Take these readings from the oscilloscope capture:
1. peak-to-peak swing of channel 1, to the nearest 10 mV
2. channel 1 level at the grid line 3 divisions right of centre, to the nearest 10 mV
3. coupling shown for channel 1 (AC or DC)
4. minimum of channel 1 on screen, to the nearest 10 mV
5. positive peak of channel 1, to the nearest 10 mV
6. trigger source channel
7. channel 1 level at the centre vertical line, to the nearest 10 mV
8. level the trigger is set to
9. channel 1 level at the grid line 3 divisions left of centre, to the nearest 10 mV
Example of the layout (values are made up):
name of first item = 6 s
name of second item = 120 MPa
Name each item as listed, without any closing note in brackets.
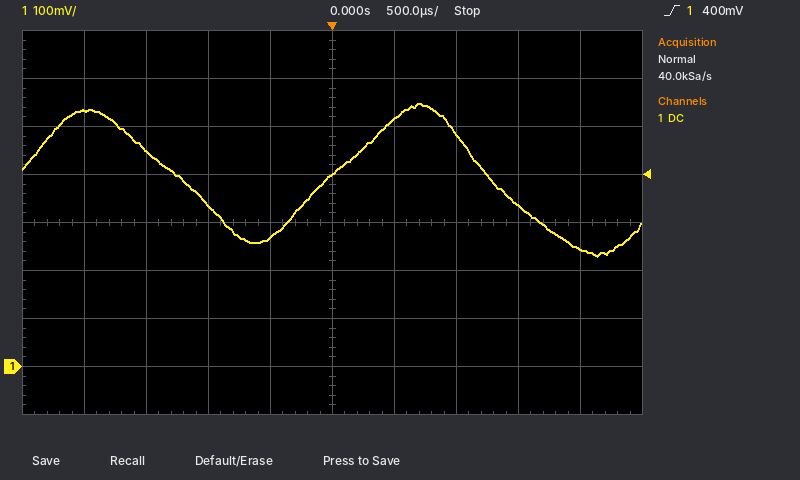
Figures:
peak-to-peak swing of channel 1, to the nearest 10 mV = 320 mV
channel 1 level at the grid line 3 divisions right of centre, to the nearest 10 mV = 340 mV
coupling shown for channel 1 = DC
minimum of channel 1 on screen, to the nearest 10 mV = 230 mV
positive peak of channel 1, to the nearest 10 mV = 550 mV
trigger source channel = channel 1
channel 1 level at the centre vertical line, to the nearest 10 mV = 400 mV
level the trigger is set to = 400 mV
channel 1 level at the grid line 3 divisions left of centre, to the nearest 10 mV = 450 mV
